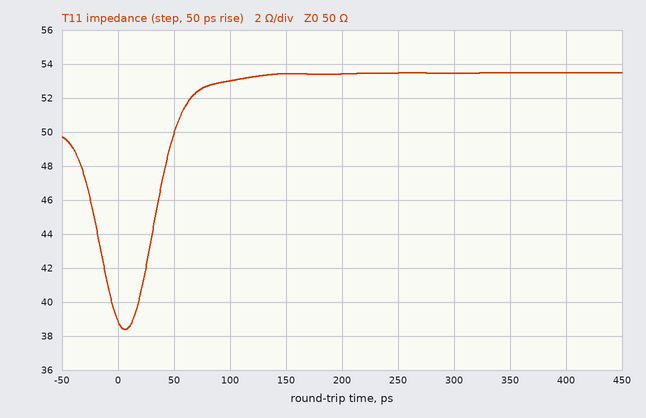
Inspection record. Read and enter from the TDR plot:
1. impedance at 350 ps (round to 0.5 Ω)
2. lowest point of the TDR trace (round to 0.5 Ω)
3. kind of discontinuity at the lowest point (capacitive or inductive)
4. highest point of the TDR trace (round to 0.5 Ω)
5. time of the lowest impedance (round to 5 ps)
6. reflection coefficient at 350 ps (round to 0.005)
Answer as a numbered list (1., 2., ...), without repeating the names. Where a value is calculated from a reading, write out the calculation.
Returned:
1. 53.5 Ω
2. 38.5 Ω
3. capacitive
4. 53.5 Ω
5. 5 ps
6. (53.5 − 50)/(53.5 + 50) ≈ +0.0338, so +0.035 to the nearest 0.005
